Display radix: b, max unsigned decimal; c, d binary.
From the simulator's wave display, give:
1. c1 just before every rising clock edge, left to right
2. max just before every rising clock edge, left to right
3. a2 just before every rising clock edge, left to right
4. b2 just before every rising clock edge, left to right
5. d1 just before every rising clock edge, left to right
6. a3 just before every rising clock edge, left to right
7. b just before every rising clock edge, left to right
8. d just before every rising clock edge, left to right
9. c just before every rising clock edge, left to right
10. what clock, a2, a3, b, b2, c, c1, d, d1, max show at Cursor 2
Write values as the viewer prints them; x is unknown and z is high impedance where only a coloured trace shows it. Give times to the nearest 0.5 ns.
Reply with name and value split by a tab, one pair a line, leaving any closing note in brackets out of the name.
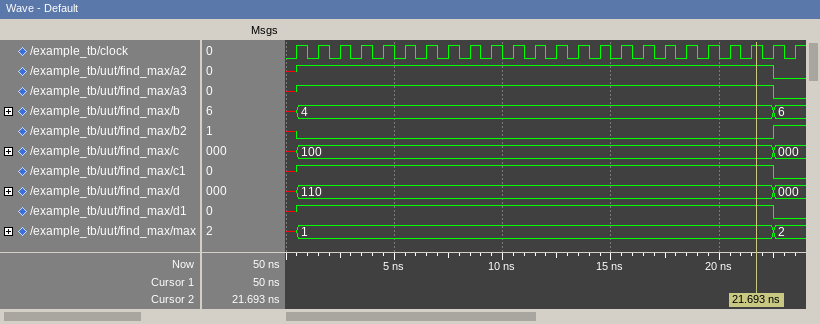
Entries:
c1 just before every rising clock edge, left to right	x 1 1 1 1 1 1 1 1 1 1 1 1 1 1 1 1 1 1 1 1 1 1 0
max just before every rising clock edge, left to right	x, 1, 1, 1, 1, 1, 1, 1, 1, 1, 1, 1, 1, 1, 1, 1, 1, 1, 1, 1, 1, 1, 1, 2
a2 just before every rising clock edge, left to right	x 1 1 1 1 1 1 1 1 1 1 1 1 1 1 1 1 1 1 1 1 1 1 0
b2 just before every rising clock edge, left to right	x 0 0 0 0 0 0 0 0 0 0 0 0 0 0 0 0 0 0 0 0 0 0 1
d1 just before every rising clock edge, left to right	x 1 1 1 1 1 1 1 1 1 1 1 1 1 1 1 1 1 1 1 1 1 1 0
a3 just before every rising clock edge, left to right	x 1 1 1 1 1 1 1 1 1 1 1 1 1 1 1 1 1 1 1 1 1 1 0
b just before every rising clock edge, left to right	x, 4, 4, 4, 4, 4, 4, 4, 4, 4, 4, 4, 4, 4, 4, 4, 4, 4, 4, 4, 4, 4, 4, 6
d just before every rising clock edge, left to right	x, 110, 110, 110, 110, 110, 110, 110, 110, 110, 110, 110, 110, 110, 110, 110, 110, 110, 110, 110, 110, 110, 110, 000
c just before every rising clock edge, left to right	x, 100, 100, 100, 100, 100, 100, 100, 100, 100, 100, 100, 100, 100, 100, 100, 100, 100, 100, 100, 100, 100, 100, 000
what clock, a2, a3, b, b2, c, c1, d, d1, max show at Cursor 2	clock=1, a2=1, a3=1, b=4, b2=0, c=100, c1=1, d=110, d1=1, max=1
